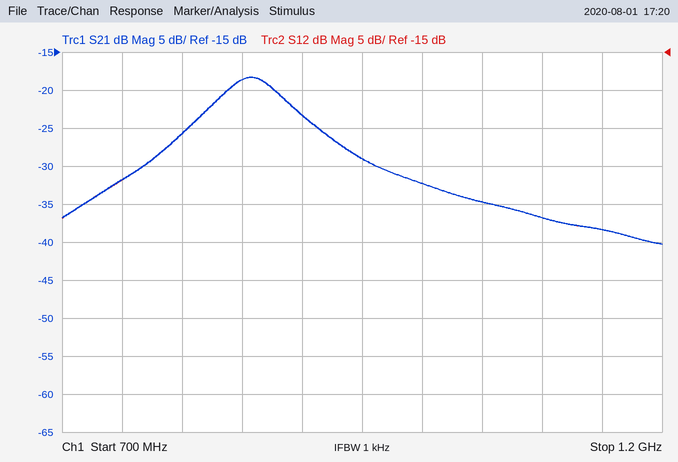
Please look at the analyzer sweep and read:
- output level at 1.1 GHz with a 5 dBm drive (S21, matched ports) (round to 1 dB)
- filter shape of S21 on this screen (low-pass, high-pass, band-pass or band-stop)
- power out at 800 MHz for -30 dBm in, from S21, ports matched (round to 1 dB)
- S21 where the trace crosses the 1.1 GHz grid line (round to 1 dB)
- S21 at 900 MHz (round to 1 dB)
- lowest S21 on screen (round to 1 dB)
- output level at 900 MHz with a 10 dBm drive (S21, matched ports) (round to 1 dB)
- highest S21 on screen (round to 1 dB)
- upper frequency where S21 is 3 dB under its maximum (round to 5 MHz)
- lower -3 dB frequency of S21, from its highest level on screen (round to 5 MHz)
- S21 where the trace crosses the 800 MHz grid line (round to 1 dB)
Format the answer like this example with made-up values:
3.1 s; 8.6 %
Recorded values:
-32 dBm; band-pass; -56 dBm; -37 dB; -23 dB; -40 dB; -13 dBm; -18 dB; 885 MHz; 830 MHz; -26 dB
